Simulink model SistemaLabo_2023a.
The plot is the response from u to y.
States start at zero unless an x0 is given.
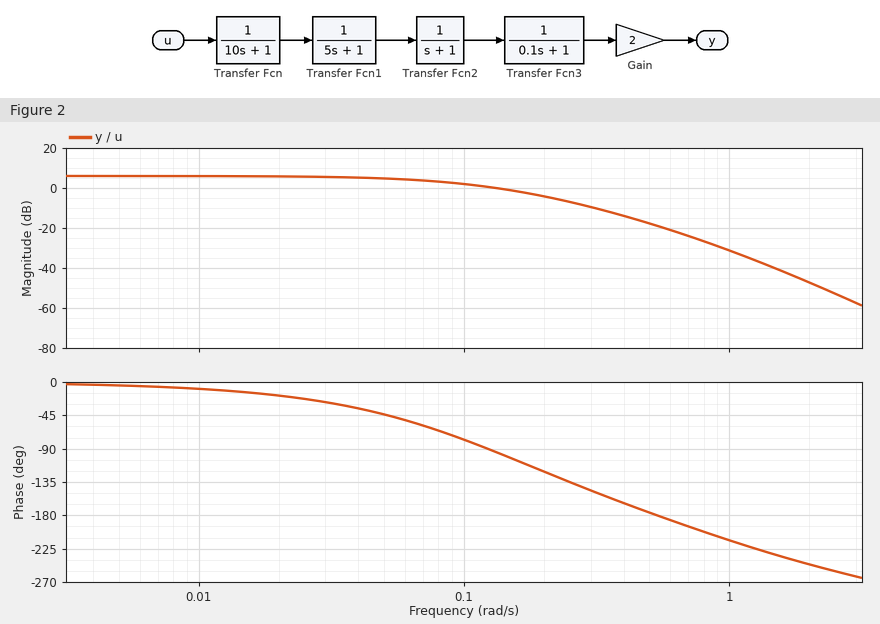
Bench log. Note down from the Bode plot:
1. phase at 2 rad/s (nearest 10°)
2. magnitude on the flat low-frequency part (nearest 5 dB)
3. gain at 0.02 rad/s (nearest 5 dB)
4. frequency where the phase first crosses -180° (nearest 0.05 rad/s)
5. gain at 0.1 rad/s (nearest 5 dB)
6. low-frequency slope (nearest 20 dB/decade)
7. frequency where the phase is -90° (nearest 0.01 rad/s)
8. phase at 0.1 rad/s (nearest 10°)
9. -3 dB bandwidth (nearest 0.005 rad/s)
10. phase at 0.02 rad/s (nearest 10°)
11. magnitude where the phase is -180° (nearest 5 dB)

-250°
5 dB
5 dB
0.55 rad/s
0 dB
0 dB/decade
0.12 rad/s
-80°
0.085 rad/s
-20°
-20 dB
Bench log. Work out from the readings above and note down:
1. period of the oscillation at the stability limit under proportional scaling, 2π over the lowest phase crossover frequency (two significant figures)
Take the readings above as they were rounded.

11 s
